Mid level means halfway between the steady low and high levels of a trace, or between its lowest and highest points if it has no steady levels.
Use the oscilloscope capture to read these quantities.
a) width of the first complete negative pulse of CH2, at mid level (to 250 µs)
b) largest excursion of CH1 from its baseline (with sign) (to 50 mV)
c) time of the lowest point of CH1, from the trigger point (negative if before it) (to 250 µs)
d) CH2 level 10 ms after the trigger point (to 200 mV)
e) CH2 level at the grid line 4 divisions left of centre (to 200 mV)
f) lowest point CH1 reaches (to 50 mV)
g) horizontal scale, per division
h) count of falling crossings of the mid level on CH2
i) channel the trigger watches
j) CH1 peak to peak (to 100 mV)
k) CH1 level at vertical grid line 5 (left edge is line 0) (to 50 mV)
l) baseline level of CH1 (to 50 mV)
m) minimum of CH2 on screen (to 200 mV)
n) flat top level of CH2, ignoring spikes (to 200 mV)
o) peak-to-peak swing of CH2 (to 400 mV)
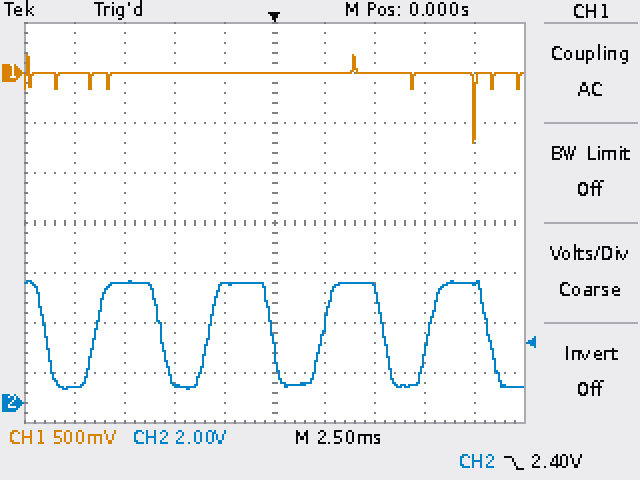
2.50 ms
-700 mV
+10.00 ms
4.8 V
600 mV
-700 mV
2.5 ms
5
CH2
900 mV
0 mV
0 mV
600 mV
4.8 V
4.4 V
